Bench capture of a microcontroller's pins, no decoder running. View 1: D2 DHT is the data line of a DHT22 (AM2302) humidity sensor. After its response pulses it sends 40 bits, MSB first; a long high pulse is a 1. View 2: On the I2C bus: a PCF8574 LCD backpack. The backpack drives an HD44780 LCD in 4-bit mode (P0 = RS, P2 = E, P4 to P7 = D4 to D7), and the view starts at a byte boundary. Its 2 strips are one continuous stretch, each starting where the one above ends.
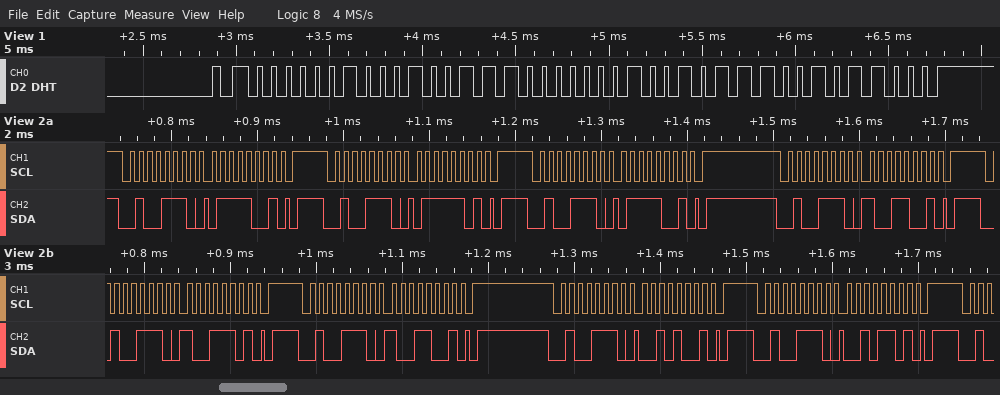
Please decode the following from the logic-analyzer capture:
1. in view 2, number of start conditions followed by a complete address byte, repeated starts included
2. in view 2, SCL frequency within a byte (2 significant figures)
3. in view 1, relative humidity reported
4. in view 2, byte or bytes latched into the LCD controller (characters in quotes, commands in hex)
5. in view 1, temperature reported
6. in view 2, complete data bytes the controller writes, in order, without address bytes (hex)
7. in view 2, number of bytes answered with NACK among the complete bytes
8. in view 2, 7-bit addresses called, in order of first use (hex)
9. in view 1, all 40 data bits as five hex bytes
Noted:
8
100 kHz
55.1 %
'y'
30.2 °C
79 7D 79 99 9D 99 29 2D
0
0x27
02 27 01 2E 58
